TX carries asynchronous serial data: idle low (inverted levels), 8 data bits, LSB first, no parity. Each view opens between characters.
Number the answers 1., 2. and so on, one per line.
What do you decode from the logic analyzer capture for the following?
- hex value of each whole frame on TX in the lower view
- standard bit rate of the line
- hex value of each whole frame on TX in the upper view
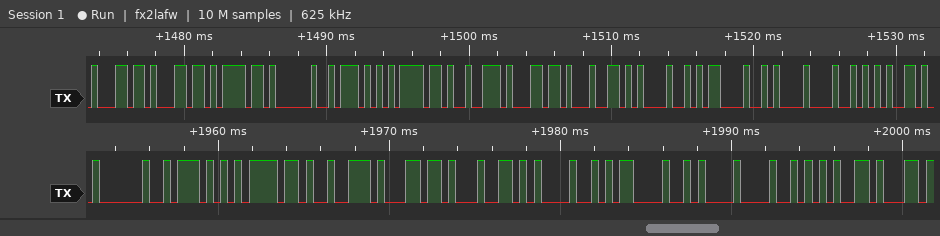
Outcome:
1. BF, 51, 21, 1B, 27, 37, BD, E5, EB, 6F, 35
2. 2400 baud
3. 27, 27, 21, BF, 51, 21, 1B, 27, 37, BD, E5, EB, 6F, 35
